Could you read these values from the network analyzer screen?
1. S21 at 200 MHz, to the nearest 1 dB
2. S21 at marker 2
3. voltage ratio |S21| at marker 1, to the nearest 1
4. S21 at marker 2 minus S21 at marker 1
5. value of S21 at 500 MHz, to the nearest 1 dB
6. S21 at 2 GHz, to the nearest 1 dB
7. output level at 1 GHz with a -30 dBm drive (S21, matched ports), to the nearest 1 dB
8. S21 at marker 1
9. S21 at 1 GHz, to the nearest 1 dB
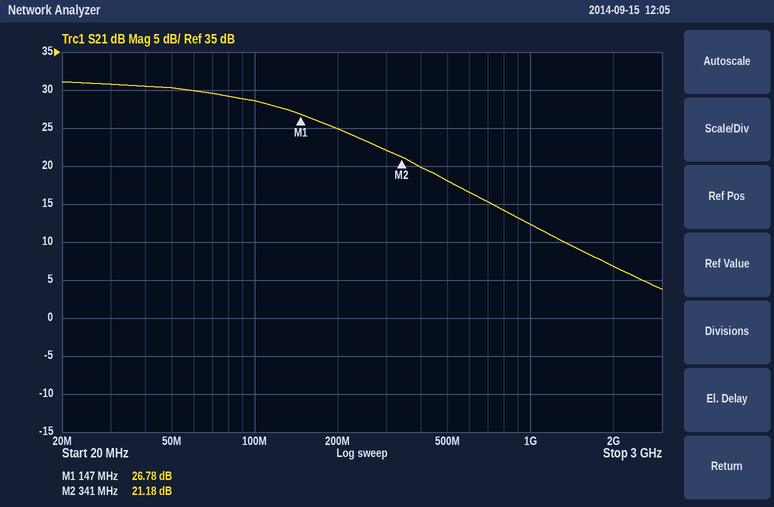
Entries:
25 dB
21.18 dB
22
-5.60 dB
18 dB
7 dB
-18 dBm
26.78 dB
12 dB
